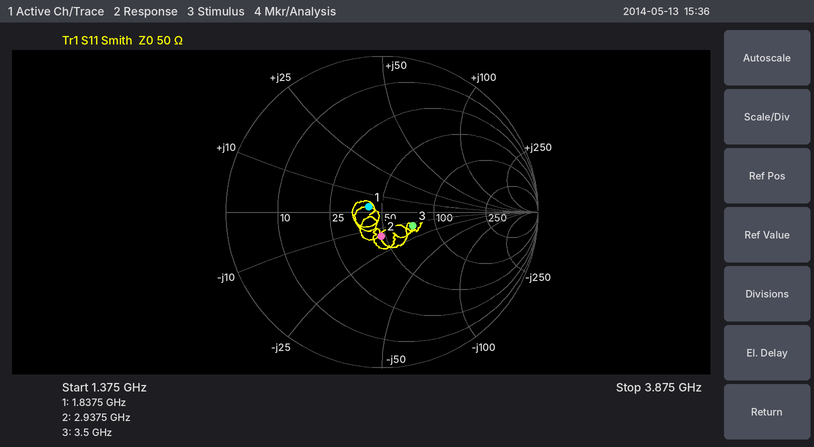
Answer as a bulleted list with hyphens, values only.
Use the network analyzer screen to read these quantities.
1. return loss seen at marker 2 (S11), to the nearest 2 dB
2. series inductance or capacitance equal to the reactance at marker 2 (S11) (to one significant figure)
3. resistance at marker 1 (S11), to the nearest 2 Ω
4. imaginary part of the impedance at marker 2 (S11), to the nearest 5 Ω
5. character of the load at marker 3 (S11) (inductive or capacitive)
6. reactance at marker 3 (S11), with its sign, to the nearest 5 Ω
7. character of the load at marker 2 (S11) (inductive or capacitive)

- 16 dB
- 4 pF
- 42 Ω
- -15 Ω
- capacitive
- -15 Ω
- capacitive
